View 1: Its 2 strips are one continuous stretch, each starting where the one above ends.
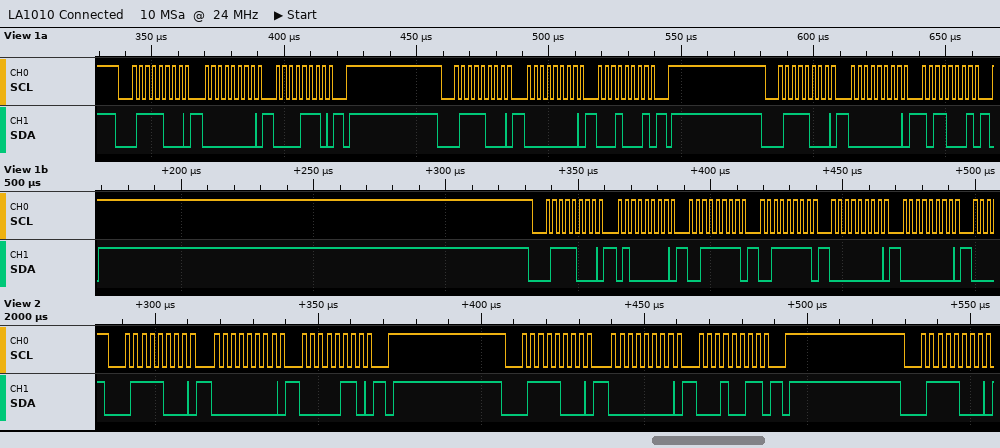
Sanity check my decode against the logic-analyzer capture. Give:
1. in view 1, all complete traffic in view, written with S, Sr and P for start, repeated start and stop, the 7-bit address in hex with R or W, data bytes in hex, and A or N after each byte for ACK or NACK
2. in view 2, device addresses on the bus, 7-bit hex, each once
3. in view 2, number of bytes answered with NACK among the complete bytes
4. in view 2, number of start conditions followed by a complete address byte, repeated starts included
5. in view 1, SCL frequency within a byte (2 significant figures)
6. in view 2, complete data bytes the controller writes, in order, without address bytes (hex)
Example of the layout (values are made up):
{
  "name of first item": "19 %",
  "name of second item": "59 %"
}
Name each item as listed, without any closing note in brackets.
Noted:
{
  "in view 1, all complete traffic in view, written with S, Sr and P for start, repeated start and stop, the 7-bit address in hex with R or W, data bytes in hex, and A or N after each byte for ACK or NACK": "S 3CW A 00 A 0E A P S 3CW A 00 A 11 A P S 3CW A 00 A B1 A P S 3CW A 40 A 3F A 3F A 00 A 00 A",
  "in view 2, device addresses on the bus, 7-bit hex, each once": "0x3C",
  "in view 2, number of bytes answered with NACK among the complete bytes": "0",
  "in view 2, number of start conditions followed by a complete address byte, repeated starts included": "3",
  "in view 1, SCL frequency within a byte": "400 kHz",
  "in view 2, complete data bytes the controller writes, in order, without address bytes": "00 06 00 13"
}
